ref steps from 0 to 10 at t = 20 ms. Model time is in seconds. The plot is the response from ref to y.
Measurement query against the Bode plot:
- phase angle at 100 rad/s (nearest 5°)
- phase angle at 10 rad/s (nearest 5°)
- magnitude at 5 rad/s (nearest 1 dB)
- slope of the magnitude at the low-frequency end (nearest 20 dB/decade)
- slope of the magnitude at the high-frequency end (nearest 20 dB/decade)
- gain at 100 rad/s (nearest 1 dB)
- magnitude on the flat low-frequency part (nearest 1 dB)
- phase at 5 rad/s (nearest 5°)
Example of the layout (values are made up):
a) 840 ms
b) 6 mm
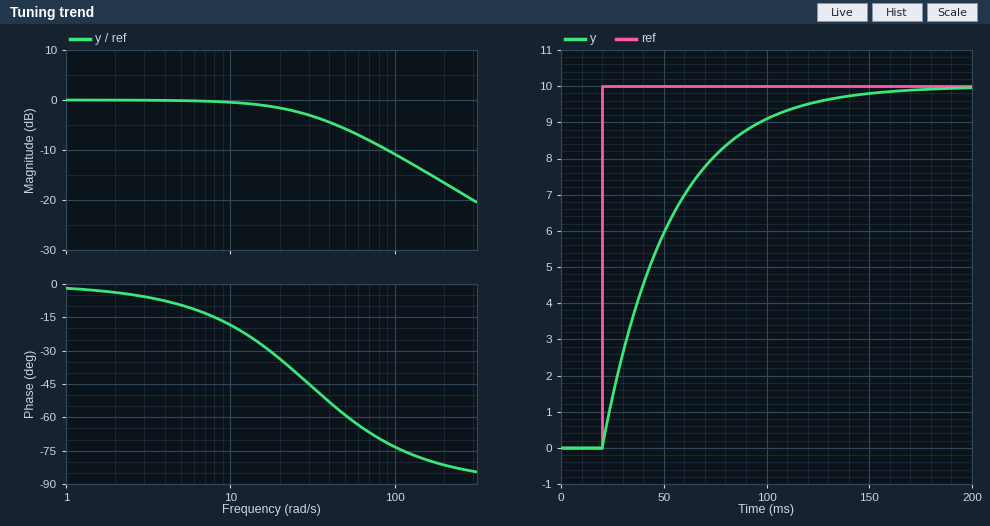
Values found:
a) -75°
b) -20°
c) 0 dB
d) 0 dB/decade
e) -20 dB/decade
f) -11 dB
g) 0 dB
h) -10°
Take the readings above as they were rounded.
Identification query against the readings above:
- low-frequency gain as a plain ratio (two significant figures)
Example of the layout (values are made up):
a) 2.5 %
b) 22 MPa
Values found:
a) 1.0
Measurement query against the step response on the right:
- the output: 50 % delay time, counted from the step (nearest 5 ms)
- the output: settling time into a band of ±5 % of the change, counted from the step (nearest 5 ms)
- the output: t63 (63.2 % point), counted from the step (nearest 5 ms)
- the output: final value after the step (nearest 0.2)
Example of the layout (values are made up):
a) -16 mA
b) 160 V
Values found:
a) 25 ms
b) 100 ms
c) 35 ms
d) 10.0
